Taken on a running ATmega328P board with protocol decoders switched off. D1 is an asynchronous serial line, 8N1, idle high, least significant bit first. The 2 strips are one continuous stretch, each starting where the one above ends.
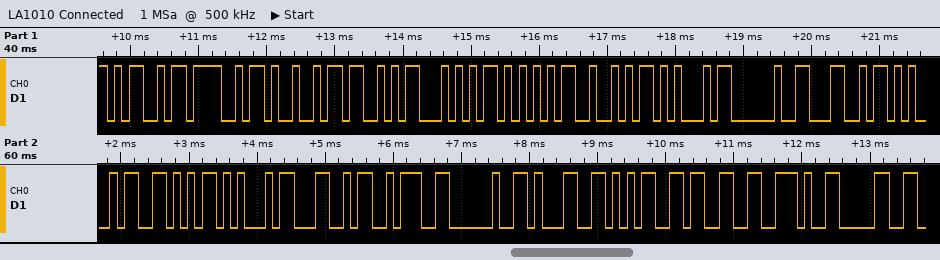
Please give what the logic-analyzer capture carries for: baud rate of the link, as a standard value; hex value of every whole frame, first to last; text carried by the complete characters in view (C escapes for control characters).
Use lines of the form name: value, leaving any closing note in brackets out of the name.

baud rate of the link, as a standard value: 9600 baud
hex value of every whole frame, first to last: 4D 4F 49 53 54 55 52 45 20 4C 45 56 45 4C 3A 20 31 35 33 2E 30
text carried by the complete characters in view: "MOISTURE LEVEL: 153.0"
